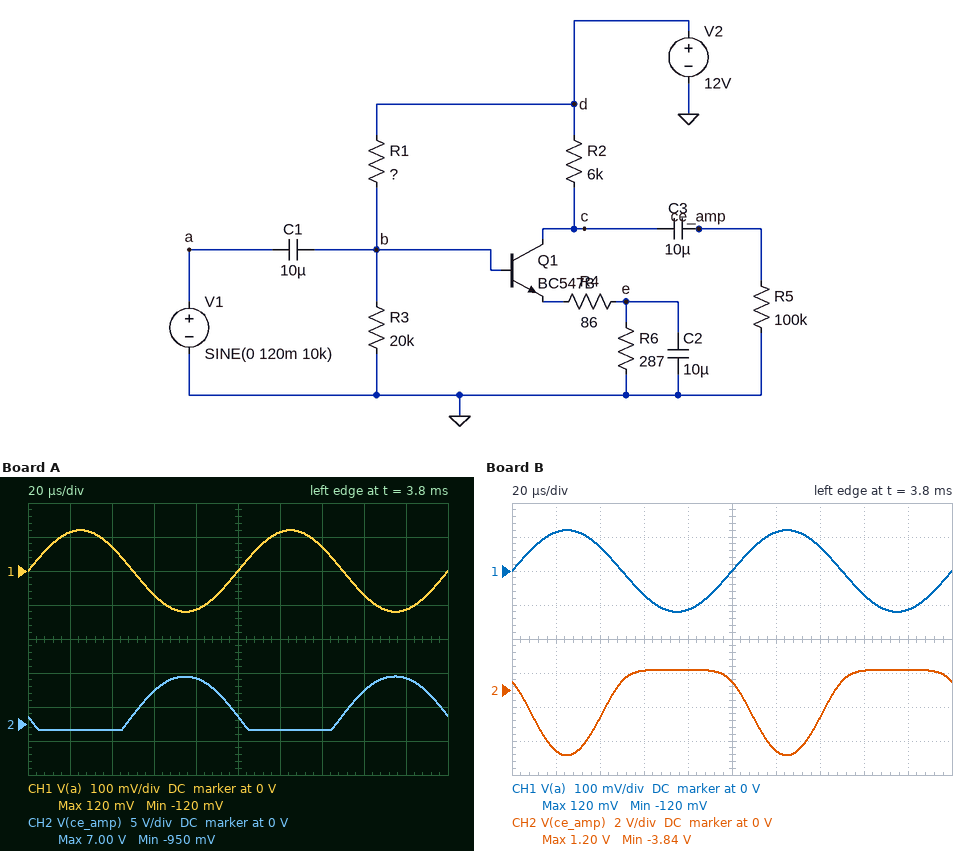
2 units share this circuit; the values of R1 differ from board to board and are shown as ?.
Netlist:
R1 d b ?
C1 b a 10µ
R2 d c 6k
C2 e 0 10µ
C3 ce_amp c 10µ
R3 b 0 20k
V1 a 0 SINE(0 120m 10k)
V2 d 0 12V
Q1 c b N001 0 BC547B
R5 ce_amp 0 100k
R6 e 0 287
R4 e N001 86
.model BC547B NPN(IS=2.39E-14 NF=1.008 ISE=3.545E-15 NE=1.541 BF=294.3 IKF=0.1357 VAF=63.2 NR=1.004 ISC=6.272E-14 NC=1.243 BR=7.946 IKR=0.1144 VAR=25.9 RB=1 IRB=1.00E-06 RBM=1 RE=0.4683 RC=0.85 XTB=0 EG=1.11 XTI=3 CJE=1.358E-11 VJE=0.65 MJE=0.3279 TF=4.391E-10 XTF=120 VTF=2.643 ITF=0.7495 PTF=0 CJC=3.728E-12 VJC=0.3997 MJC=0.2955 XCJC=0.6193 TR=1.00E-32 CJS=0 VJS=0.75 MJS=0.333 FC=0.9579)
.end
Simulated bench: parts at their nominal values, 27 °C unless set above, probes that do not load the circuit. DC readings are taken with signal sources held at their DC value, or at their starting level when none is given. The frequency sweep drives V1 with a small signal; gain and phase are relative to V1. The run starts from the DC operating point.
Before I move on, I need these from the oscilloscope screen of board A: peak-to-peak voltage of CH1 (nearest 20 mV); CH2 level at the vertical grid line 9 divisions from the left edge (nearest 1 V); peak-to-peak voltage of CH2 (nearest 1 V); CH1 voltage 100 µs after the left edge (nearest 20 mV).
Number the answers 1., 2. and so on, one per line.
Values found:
1. 240 mV
2. 7 V
3. 8 V
4. 0 V
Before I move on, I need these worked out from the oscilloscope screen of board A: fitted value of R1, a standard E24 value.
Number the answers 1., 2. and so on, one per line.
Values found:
1. 150 kΩ
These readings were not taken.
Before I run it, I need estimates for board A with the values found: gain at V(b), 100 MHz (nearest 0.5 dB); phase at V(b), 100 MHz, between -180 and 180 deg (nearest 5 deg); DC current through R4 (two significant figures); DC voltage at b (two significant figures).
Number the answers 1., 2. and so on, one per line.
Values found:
1. 0 dB
2. 0 deg
3. 1.7 mA
4. 1.3 V
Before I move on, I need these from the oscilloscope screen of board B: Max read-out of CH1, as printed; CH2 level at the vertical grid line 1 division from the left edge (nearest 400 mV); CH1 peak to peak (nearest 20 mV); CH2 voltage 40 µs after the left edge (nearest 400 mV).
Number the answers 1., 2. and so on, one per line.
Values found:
1. 120 mV
2. -3.6 V
3. 240 mV
4. -1.6 V
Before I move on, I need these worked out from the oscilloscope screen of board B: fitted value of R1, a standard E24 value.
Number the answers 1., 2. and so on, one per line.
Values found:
1. 330 kΩ
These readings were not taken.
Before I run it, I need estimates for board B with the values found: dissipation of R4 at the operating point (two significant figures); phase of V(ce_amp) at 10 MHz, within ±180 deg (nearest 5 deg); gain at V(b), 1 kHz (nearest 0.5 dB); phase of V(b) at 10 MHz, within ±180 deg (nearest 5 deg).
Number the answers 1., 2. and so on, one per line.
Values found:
1. 3.9 µW
2. 145 deg
3. 0 dB
4. 0 deg
